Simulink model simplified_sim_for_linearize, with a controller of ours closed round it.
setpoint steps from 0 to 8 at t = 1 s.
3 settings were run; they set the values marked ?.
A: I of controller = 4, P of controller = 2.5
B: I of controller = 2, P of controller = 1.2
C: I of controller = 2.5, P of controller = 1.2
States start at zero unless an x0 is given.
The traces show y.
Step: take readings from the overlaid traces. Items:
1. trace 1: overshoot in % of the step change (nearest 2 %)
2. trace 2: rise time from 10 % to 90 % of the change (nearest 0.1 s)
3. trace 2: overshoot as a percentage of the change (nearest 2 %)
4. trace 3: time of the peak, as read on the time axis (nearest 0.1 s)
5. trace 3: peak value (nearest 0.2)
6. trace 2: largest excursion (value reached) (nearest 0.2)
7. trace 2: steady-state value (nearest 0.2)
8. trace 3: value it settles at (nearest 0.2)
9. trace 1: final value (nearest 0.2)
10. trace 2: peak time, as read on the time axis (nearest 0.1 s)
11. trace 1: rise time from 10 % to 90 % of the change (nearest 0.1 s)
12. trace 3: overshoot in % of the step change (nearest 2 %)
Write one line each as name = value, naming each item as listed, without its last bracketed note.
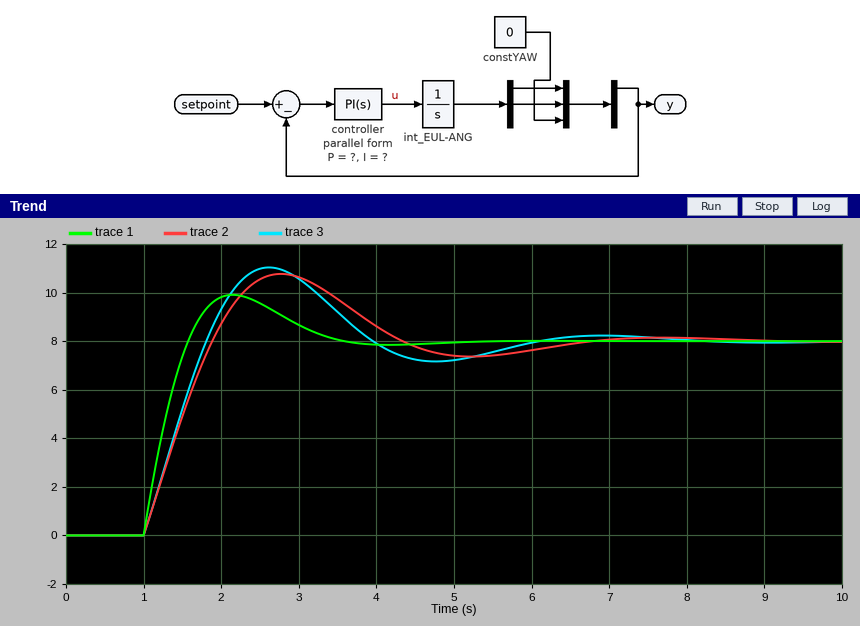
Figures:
trace 1: overshoot in % of the step change = 24 %
trace 2: rise time from 10 % to 90 % of the change = 0.7 s
trace 2: overshoot as a percentage of the change = 34 %
trace 3: time of the peak, as read on the time axis = 2.6 s
trace 3: peak value = 11.0
trace 2: largest excursion (value reached) = 10.8
trace 2: steady-state value = 8.0
trace 3: value it settles at = 8.0
trace 1: final value = 8.0
trace 2: peak time, as read on the time axis = 2.8 s
trace 1: rise time from 10 % to 90 % of the change = 0.4 s
trace 3: overshoot in % of the step change = 38 %
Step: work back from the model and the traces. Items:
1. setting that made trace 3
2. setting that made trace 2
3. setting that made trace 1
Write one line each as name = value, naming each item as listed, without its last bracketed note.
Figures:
setting that made trace 3 = C
setting that made trace 2 = B
setting that made trace 1 = A
